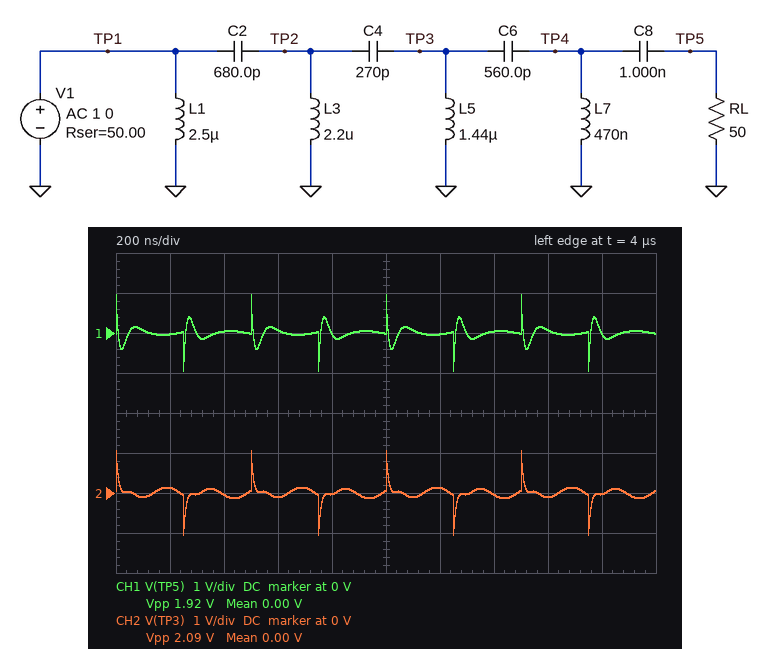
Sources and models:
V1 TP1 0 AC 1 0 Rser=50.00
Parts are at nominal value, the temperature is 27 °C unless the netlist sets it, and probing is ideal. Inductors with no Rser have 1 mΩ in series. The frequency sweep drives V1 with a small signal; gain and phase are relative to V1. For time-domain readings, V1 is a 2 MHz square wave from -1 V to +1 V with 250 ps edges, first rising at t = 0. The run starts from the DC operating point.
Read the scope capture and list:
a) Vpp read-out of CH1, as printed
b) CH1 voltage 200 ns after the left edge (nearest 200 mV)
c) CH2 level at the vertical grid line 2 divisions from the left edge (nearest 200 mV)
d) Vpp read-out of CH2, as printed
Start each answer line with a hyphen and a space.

- 1.92 V
- 0 V
- 0 V
- 2.09 V
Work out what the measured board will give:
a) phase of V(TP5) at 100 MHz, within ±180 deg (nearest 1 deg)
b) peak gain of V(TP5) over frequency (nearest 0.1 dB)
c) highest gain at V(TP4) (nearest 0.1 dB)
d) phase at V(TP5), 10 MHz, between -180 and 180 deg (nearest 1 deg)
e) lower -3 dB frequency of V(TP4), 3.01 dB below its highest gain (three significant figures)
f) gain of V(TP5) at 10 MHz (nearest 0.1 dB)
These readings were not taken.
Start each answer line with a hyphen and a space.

- 16 deg
- -6.0 dB
- -5.3 dB
- 162 deg
- 4.10 MHz
- -9.4 dB
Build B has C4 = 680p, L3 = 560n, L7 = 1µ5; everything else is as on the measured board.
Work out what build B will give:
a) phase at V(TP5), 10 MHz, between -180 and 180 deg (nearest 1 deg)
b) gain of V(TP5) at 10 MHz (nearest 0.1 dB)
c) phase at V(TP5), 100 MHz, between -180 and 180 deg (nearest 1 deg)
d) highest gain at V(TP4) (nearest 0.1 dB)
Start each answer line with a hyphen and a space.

- 131 deg
- -7.1 dB
- 13 deg
- -6.0 dB
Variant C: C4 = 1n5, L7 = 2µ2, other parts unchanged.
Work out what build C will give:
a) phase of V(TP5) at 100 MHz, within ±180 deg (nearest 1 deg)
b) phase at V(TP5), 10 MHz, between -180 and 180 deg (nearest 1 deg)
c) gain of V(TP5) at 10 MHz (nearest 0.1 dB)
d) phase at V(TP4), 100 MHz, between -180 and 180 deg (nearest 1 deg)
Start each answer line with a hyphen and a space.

- 9 deg
- 92 deg
- -6.2 dB
- 7 deg
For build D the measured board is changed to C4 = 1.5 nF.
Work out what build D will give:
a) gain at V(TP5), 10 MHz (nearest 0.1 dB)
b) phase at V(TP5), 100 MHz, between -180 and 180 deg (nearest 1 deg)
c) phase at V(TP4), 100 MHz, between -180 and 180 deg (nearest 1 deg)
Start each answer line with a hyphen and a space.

- -7.1 dB
- 13 deg
- 11 deg
